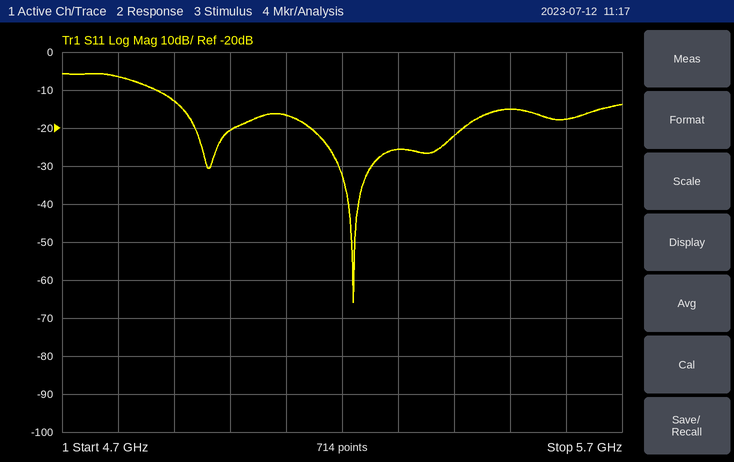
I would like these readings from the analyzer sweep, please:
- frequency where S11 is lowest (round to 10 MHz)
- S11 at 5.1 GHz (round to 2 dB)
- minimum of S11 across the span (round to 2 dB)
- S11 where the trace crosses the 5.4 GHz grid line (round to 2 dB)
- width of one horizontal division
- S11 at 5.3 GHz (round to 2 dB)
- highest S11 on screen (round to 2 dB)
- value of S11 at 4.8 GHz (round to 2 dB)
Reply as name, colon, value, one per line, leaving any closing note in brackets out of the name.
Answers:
frequency where S11 is lowest: 5.22 GHz
S11 at 5.1 GHz: -16 dB
minimum of S11 across the span: -66 dB
S11 where the trace crosses the 5.4 GHz grid line: -22 dB
width of one horizontal division: 100 MHz
S11 at 5.3 GHz: -26 dB
highest S11 on screen: -6 dB
value of S11 at 4.8 GHz: -6 dB
